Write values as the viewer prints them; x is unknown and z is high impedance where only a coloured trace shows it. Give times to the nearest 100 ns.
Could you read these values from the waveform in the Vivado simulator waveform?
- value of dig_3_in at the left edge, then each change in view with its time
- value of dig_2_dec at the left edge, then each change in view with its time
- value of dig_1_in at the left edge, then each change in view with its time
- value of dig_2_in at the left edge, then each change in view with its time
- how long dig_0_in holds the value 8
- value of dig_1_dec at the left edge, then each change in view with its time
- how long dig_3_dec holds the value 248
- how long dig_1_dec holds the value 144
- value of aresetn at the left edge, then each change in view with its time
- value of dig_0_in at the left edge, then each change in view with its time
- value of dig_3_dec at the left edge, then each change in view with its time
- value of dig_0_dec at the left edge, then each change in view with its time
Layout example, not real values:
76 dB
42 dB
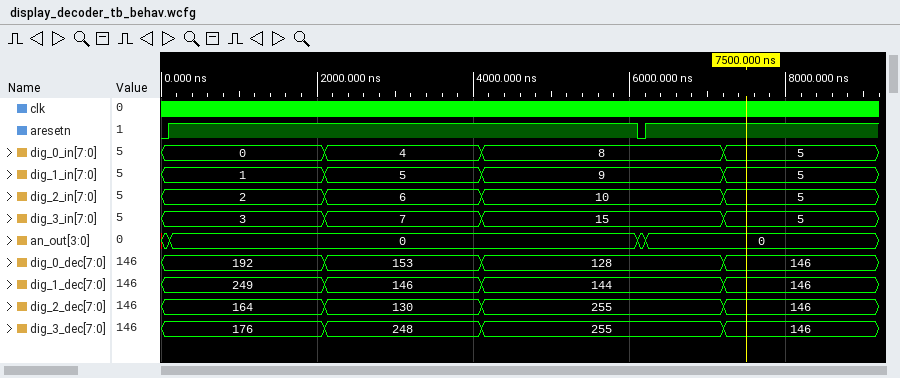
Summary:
3, 7 at 2100 ns, 15 at 4100 ns, 5 at 7200 ns
164, 130 at 2100 ns, 255 at 4100 ns, 146 at 7200 ns
1, 5 at 2100 ns, 9 at 4100 ns, 5 at 7200 ns
2, 6 at 2100 ns, 10 at 4100 ns, 5 at 7200 ns
3100 ns
249, 146 at 2100 ns, 144 at 4100 ns, 146 at 7200 ns
2000 ns
3100 ns
0, 1 at 100 ns, 0 at 6100 ns, 1 at 6200 ns
0, 4 at 2100 ns, 8 at 4100 ns, 5 at 7200 ns
176, 248 at 2100 ns, 255 at 4100 ns, 146 at 7200 ns
192, 153 at 2100 ns, 128 at 4100 ns, 146 at 7200 ns
